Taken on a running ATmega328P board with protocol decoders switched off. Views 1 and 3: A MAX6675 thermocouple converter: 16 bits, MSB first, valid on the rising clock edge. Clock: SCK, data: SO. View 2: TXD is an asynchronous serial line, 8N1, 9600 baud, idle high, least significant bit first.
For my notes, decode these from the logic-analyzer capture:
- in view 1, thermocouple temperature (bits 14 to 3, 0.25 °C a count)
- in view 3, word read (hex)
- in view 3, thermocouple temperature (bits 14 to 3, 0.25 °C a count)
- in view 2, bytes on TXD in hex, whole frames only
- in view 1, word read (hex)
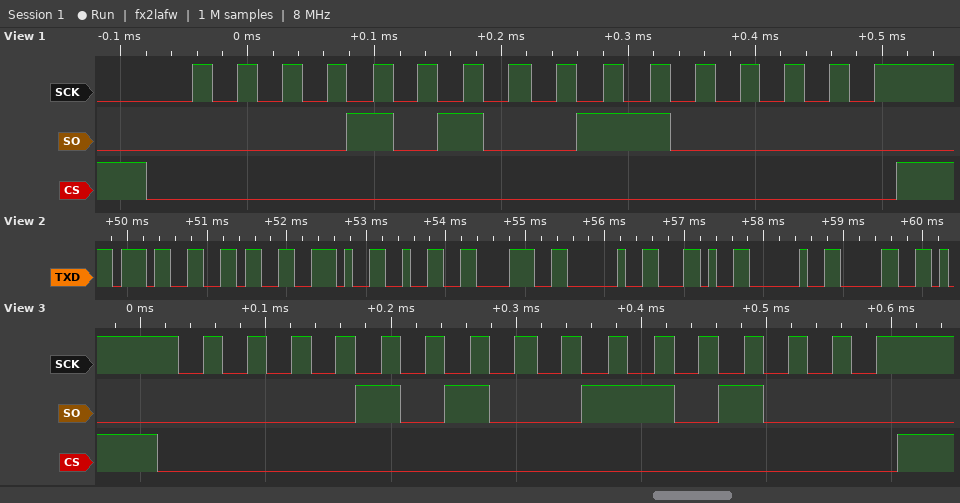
83.00 °C
0x0A68
83.25 °C
37 36 2E 32 38 20 2C 20 30
0x0A60
